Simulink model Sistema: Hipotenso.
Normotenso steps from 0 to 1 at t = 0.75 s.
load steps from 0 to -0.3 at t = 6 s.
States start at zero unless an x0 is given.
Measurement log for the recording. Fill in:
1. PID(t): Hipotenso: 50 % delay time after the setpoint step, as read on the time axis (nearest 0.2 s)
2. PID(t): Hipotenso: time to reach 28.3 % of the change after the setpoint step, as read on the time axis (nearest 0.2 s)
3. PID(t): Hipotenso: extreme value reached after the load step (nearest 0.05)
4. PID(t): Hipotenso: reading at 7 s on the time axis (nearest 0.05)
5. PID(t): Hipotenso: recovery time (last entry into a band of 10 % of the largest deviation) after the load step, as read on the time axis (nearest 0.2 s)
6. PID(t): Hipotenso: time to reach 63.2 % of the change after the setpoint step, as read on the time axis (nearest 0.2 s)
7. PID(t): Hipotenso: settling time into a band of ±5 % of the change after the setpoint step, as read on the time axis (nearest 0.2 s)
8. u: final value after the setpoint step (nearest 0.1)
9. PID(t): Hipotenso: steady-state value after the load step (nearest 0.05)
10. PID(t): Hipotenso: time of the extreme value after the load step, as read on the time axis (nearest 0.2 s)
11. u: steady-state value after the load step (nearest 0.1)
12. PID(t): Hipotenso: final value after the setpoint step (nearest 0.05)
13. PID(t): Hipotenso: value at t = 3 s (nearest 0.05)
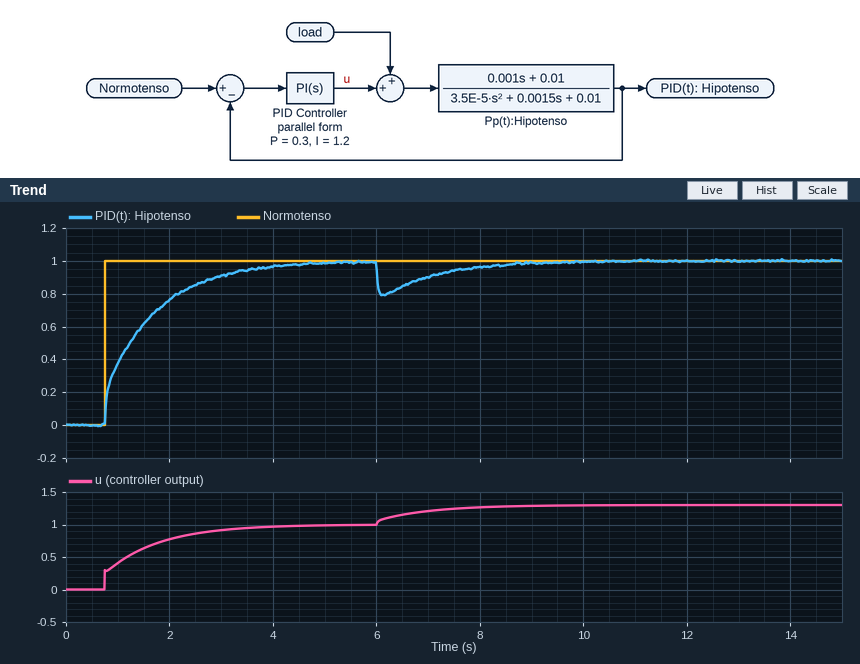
1.2 s
0.8 s
0.80
0.90
8.6 s
1.6 s
3.6 s
1.0
1.00
6.2 s
1.3
1.00
0.90
